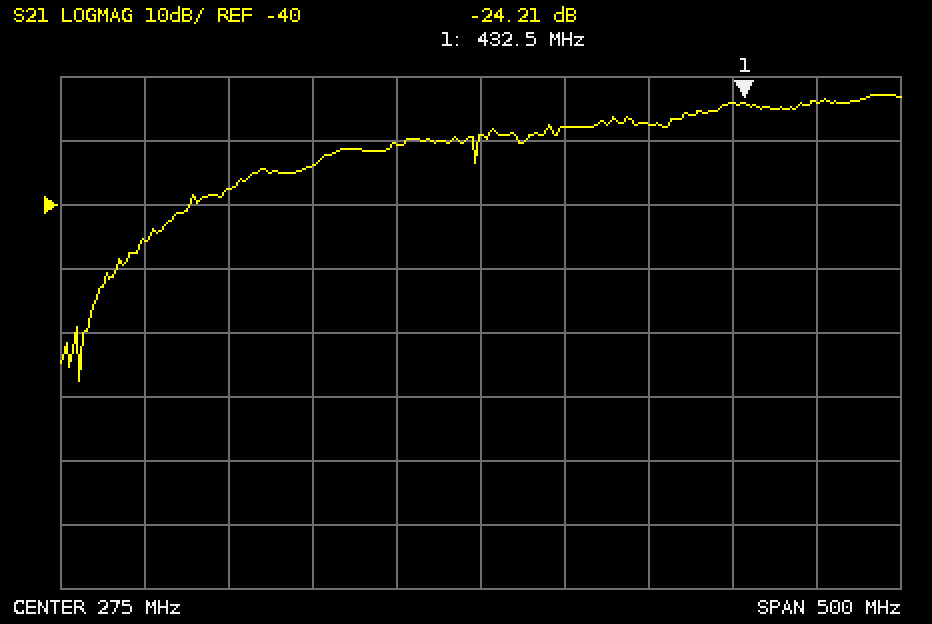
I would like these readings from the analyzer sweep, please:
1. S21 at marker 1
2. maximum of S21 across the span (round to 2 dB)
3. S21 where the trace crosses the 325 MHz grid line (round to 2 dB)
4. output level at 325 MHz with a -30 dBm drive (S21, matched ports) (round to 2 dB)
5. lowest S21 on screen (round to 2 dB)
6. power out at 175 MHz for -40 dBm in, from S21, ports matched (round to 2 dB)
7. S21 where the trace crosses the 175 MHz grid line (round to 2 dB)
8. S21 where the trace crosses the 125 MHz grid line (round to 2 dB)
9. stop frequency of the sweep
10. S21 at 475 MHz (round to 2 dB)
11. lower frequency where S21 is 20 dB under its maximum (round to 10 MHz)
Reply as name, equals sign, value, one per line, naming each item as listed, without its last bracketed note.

S21 at marker 1 = -24.21 dB
maximum of S21 across the span = -22 dB
S21 where the trace crosses the 325 MHz grid line = -28 dB
output level at 325 MHz with a -30 dBm drive (S21, matched ports) = -58 dBm
lowest S21 on screen = -68 dB
power out at 175 MHz for -40 dBm in, from S21, ports matched = -74 dBm
S21 where the trace crosses the 175 MHz grid line = -34 dB
S21 where the trace crosses the 125 MHz grid line = -38 dB
stop frequency of the sweep = 525 MHz
S21 at 475 MHz = -24 dB
lower frequency where S21 is 20 dB under its maximum = 90 MHz
